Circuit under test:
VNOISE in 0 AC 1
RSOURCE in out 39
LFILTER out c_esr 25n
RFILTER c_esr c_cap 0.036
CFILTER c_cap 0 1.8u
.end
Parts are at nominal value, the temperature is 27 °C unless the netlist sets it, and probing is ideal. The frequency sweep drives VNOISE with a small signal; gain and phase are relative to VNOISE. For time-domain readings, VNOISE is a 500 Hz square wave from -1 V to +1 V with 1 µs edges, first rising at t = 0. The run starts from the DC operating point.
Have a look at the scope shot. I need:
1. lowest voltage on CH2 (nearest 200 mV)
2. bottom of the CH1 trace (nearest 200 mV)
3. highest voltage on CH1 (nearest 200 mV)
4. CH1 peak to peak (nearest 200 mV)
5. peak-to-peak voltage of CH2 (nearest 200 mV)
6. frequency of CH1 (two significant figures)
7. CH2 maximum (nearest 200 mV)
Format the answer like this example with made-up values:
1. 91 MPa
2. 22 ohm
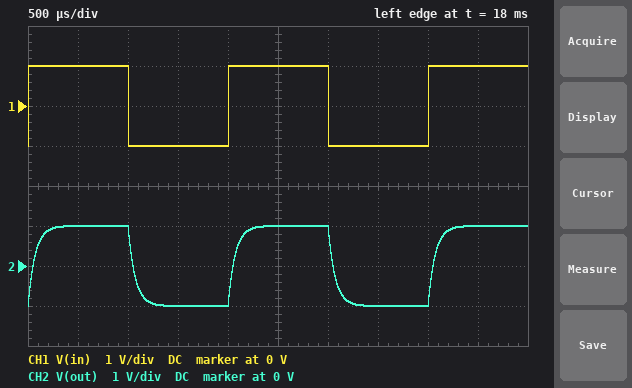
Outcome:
1. -1.0 V
2. -1.0 V
3. 1.0 V
4. 2.0 V
5. 2.0 V
6. 500 Hz
7. 1.0 V
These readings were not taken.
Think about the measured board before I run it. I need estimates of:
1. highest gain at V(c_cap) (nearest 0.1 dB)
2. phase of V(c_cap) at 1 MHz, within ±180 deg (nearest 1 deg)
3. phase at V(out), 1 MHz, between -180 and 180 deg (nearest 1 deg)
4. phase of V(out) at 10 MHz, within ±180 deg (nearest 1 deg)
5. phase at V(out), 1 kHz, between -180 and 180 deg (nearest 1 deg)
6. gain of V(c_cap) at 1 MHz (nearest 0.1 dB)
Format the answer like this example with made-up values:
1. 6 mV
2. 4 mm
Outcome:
1. 0 dB
2. -90 deg
3. 62 deg
4. 86 deg
5. -24 deg
6. -52.9 dB
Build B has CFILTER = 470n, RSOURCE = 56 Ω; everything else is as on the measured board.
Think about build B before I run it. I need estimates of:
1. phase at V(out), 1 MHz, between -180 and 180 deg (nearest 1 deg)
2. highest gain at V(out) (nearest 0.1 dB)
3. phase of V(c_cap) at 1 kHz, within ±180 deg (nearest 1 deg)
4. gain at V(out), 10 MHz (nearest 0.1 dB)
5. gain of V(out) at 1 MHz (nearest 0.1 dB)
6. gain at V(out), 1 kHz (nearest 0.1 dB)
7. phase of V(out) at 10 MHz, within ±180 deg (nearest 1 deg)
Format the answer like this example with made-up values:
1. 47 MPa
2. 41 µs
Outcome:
1. -79 deg
2. 0 dB
3. -9 deg
4. -31.2 dB
5. -49.6 dB
6. -0.1 dB
7. 87 deg
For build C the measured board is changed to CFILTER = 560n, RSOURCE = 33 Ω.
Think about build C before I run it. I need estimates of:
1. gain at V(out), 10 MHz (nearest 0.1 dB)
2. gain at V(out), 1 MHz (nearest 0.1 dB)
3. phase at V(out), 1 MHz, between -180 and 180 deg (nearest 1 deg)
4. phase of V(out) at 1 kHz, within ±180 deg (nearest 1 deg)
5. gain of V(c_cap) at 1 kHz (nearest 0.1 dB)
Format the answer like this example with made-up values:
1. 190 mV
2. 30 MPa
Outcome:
1. -26.6 dB
2. -48.0 dB
3. -74 deg
4. -7 deg
5. -0.1 dB
